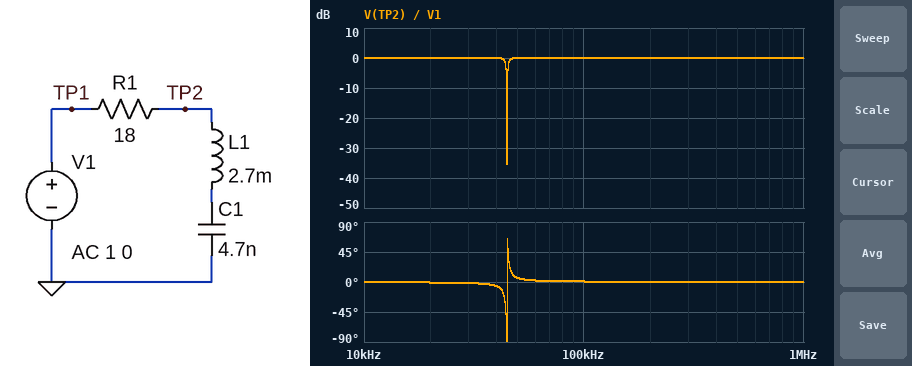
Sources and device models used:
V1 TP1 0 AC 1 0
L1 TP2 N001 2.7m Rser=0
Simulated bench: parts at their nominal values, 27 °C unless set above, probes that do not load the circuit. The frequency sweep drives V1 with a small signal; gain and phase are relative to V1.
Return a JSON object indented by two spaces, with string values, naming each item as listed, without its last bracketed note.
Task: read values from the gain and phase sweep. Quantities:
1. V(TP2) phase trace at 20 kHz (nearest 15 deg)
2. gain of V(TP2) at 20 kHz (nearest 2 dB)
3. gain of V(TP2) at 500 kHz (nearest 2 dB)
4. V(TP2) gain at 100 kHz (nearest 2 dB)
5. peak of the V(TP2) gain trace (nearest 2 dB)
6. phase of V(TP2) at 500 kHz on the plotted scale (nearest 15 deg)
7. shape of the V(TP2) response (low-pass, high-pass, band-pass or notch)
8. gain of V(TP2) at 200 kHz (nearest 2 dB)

{
  "V(TP2) phase trace at 20 kHz": "0 deg",
  "gain of V(TP2) at 20 kHz": "0 dB",
  "gain of V(TP2) at 500 kHz": "0 dB",
  "V(TP2) gain at 100 kHz": "0 dB",
  "peak of the V(TP2) gain trace": "0 dB",
  "phase of V(TP2) at 500 kHz on the plotted scale": "0 deg",
  "shape of the V(TP2) response": "notch",
  "gain of V(TP2) at 200 kHz": "0 dB"
}
